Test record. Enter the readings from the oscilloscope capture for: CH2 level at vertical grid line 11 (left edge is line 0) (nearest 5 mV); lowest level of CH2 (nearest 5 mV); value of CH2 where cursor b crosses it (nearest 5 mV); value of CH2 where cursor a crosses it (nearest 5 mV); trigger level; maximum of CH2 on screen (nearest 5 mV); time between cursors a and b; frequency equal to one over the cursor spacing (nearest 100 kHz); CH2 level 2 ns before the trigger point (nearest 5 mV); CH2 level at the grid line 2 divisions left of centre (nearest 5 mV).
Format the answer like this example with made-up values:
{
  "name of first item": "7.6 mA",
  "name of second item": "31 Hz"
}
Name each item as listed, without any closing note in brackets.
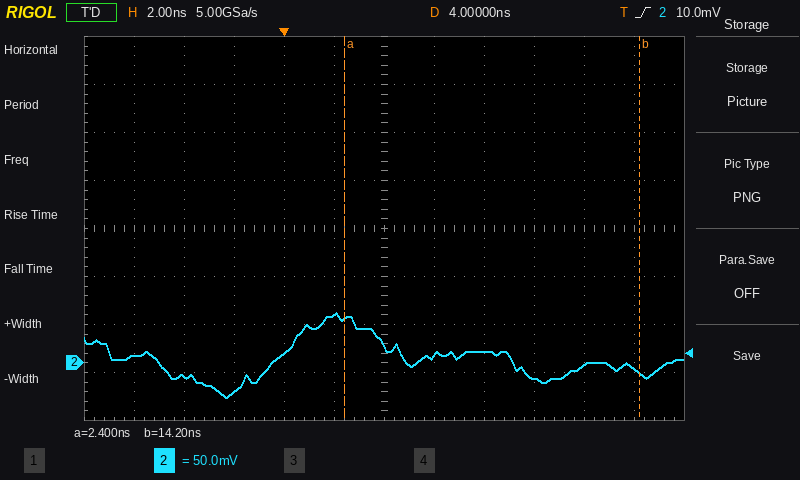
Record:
{
  "CH2 level at vertical grid line 11 (left edge is line 0)": "-5 mV",
  "lowest level of CH2": "-35 mV",
  "value of CH2 where cursor b crosses it": "-10 mV",
  "value of CH2 where cursor a crosses it": "45 mV",
  "trigger level": "10.0 mV",
  "maximum of CH2 on screen": "50 mV",
  "time between cursors a and b": "11.8 ns",
  "frequency equal to one over the cursor spacing": "84.7 MHz",
  "CH2 level 2 ns before the trigger point": "-30 mV",
  "CH2 level at the grid line 2 divisions left of centre": "10 mV"
}
